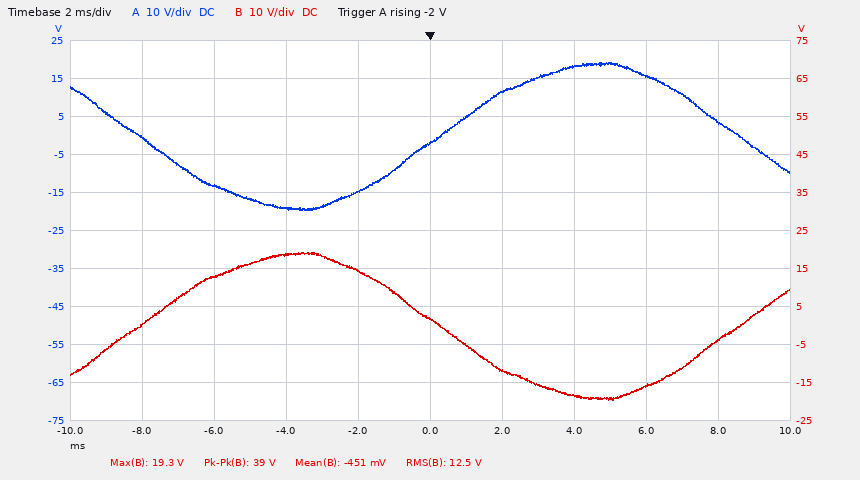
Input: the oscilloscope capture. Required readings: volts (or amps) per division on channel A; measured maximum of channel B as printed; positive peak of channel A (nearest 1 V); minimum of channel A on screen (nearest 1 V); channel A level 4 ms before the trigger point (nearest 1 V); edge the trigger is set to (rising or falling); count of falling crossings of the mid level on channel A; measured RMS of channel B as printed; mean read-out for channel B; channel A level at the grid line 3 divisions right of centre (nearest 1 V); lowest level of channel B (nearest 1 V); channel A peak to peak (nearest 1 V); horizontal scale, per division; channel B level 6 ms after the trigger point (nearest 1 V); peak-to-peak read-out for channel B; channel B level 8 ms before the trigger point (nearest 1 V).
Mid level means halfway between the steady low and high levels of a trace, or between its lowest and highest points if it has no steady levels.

10 V
19.3 V
19 V
-20 V
-19 V
rising
2
12.5 V
-451 mV
16 V
-20 V
39 V
2 ms
-16 V
39 V
0 V
